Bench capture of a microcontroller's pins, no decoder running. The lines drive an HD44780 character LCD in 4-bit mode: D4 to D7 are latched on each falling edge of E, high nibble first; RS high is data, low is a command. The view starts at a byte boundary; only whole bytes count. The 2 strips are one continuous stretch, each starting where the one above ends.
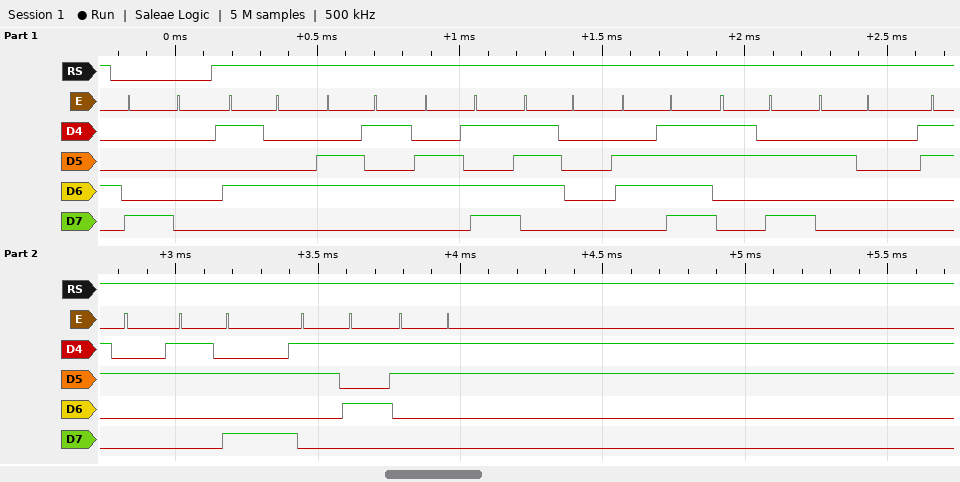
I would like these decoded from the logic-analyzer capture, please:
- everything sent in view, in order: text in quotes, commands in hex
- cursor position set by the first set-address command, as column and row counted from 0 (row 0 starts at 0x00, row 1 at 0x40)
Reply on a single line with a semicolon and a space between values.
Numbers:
0x80 "Tempo: 2:53"; column 0, row 0
